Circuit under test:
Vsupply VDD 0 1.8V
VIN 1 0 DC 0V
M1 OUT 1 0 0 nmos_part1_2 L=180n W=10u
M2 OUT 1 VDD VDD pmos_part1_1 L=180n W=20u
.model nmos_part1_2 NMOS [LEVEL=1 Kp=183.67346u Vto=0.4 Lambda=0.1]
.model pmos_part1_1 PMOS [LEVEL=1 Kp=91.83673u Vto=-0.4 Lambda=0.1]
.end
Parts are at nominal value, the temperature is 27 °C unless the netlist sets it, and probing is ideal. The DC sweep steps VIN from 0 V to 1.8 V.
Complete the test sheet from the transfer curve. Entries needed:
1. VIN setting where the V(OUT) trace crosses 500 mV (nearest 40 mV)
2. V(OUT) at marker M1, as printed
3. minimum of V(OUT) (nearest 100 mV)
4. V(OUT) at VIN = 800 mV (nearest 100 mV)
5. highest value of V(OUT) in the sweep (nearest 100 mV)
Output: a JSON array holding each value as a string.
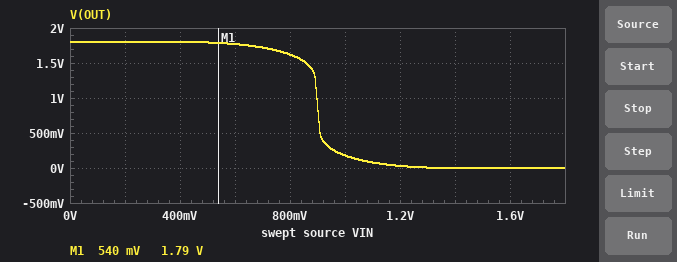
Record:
["920 mV", "1.79 V", "0 V", "1.6 V", "1.8 V"]
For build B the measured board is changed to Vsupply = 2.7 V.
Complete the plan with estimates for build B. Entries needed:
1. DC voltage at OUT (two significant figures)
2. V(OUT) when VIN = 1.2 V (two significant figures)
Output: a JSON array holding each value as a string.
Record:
["2.7 V", "2.3 V"]
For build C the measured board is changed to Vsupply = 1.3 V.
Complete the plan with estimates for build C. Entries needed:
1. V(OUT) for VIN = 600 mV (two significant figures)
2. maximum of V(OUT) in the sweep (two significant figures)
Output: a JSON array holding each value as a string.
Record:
["1.2 V", "1.3 V"]
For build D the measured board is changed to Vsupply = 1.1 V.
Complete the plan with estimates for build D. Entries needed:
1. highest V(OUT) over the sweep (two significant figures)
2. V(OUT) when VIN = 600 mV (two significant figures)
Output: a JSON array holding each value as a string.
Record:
["1.1 V", "30 mV"]
